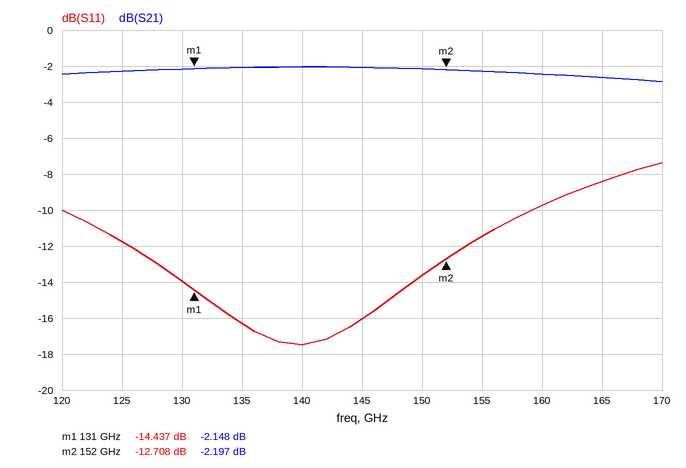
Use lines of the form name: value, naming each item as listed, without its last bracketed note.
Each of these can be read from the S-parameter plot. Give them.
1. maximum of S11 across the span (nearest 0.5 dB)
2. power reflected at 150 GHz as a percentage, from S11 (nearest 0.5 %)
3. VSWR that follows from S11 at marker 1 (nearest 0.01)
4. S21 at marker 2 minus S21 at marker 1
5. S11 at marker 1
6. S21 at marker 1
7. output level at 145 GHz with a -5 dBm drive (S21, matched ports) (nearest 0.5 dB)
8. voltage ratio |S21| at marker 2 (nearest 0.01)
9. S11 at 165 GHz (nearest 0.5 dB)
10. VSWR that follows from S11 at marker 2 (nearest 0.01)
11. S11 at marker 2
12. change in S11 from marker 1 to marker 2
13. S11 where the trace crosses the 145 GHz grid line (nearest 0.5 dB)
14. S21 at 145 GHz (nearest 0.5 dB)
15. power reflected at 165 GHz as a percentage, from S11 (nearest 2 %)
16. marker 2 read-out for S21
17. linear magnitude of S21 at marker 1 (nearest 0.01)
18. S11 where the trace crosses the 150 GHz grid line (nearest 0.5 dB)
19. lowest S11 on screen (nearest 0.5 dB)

maximum of S11 across the span: -7.5 dB
power reflected at 150 GHz as a percentage, from S11: 4.5 %
VSWR that follows from S11 at marker 1: 1.47
S21 at marker 2 minus S21 at marker 1: -0.049 dB
S11 at marker 1: -14.437 dB
S21 at marker 1: -2.148 dB
output level at 145 GHz with a -5 dBm drive (S21, matched ports): -7.0 dBm
voltage ratio |S21| at marker 2: 0.78
S11 at 165 GHz: -8.5 dB
VSWR that follows from S11 at marker 2: 1.60
S11 at marker 2: -12.708 dB
change in S11 from marker 1 to marker 2: 1.729 dB
S11 where the trace crosses the 145 GHz grid line: -16.0 dB
S21 at 145 GHz: -2.0 dB
power reflected at 165 GHz as a percentage, from S11: 14 %
marker 2 read-out for S21: -2.197 dB
linear magnitude of S21 at marker 1: 0.78
S11 where the trace crosses the 150 GHz grid line: -13.5 dB
lowest S11 on screen: -17.5 dB
